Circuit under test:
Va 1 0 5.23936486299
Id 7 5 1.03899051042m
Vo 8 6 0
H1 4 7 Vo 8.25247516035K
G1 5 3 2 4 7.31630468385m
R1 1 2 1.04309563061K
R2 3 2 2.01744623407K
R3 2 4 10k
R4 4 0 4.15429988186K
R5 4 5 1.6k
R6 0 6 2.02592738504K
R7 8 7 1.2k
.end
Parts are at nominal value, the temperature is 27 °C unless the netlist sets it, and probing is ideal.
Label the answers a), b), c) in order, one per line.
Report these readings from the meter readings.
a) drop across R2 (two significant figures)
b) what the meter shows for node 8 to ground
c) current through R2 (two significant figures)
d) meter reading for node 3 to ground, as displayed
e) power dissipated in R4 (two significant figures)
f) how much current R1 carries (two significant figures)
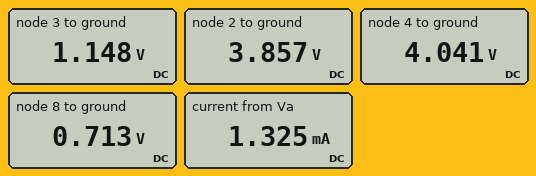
a) 2.7 V
b) 0.713 V
c) 1.3 mA
d) 1.148 V
e) 3.9 mW
f) 1.3 mA
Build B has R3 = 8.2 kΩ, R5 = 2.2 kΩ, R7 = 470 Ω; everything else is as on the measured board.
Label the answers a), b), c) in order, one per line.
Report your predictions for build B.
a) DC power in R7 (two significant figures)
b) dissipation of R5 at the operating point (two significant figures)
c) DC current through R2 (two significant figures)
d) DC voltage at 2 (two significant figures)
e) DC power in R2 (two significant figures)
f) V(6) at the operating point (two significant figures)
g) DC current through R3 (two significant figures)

a) 66 µW
b) 13 mW
c) 1.4 mA
d) 3.8 V
e) 3.8 mW
f) 760 mV
g) 23 µA
